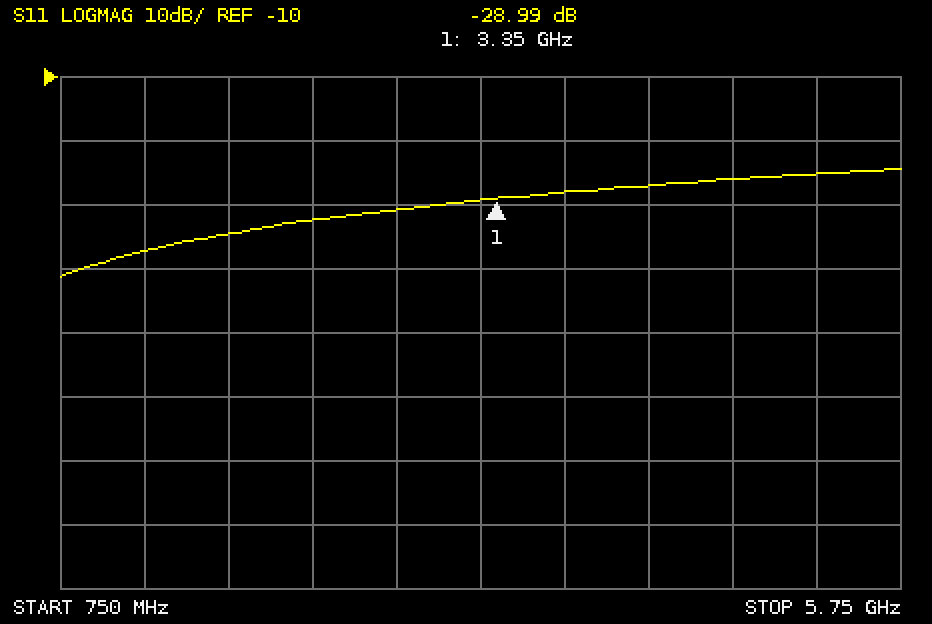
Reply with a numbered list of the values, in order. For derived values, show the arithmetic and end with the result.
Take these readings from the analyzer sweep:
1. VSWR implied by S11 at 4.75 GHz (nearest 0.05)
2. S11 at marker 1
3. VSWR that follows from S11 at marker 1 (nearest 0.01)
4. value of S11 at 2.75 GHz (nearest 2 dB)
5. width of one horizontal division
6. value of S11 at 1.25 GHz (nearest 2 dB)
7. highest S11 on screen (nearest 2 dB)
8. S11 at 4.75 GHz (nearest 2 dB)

1. |Γ| = 10^(-26/20) = 0.0501; VSWR = (1 + 0.0501)/(1 − 0.0501) ≈ 1.11, so 1.10 to the nearest 0.05
2. -28.99 dB
3. (1 + 0.0355)/(1 − 0.0355) ≈ 1.07
4. -30 dB
5. 500 MHz
6. -38 dB
7. -24 dB
8. -26 dB
